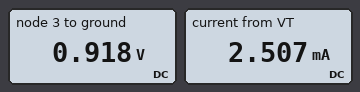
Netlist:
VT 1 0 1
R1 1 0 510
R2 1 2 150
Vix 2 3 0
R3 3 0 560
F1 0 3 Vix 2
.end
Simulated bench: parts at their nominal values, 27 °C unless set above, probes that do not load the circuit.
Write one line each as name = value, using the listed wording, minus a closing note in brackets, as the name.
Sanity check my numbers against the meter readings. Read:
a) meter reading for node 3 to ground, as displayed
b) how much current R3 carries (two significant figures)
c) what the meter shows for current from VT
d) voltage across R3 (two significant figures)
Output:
meter reading for node 3 to ground, as displayed = 0.918 V
how much current R3 carries = 1.6 mA
what the meter shows for current from VT = 2.507 mA
voltage across R3 = 920 mV
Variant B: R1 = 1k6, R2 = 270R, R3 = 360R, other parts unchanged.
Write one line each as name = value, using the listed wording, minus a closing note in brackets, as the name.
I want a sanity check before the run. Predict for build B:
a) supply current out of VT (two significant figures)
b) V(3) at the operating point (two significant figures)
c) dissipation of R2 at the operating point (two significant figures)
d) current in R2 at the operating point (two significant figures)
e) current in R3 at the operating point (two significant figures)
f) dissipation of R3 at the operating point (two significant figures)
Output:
supply current out of VT = 1.4 mA
V(3) at the operating point = 800 mV
dissipation of R2 at the operating point = 150 µW
current in R2 at the operating point = 740 µA
current in R3 at the operating point = 2.2 mA
dissipation of R3 at the operating point = 1.8 mW
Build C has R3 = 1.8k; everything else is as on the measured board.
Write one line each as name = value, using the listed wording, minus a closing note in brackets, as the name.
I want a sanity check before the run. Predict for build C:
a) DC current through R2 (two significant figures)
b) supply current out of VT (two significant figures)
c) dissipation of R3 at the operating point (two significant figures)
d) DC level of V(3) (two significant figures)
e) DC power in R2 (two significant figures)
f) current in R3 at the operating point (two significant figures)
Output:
DC current through R2 = 180 µA
supply current out of VT = 2.1 mA
dissipation of R3 at the operating point = 530 µW
DC level of V(3) = 970 mV
DC power in R2 = 4.9 µW
current in R3 at the operating point = 540 µA
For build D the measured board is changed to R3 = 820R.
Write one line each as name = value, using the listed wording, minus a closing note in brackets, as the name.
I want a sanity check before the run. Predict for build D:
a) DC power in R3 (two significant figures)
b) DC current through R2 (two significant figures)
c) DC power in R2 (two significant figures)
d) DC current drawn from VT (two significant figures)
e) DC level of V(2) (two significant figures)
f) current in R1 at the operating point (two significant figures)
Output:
DC power in R3 = 1.1 mW
DC current through R2 = 380 µA
DC power in R2 = 22 µW
DC current drawn from VT = 2.3 mA
DC level of V(2) = 940 mV
current in R1 at the operating point = 2.0 mA
